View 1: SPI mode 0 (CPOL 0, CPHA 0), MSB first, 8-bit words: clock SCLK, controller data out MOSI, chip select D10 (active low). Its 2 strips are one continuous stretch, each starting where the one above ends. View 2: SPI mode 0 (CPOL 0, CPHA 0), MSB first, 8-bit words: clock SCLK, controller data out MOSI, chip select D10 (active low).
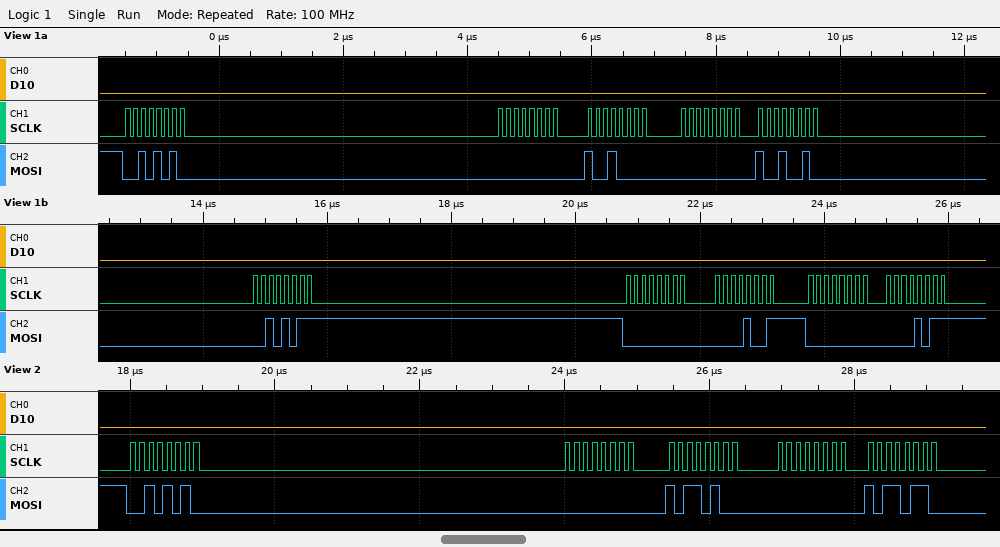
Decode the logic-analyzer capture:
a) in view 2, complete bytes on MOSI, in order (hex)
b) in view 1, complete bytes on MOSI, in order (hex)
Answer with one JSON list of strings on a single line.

["2A 00 B4 00 B6", "0x2A 0x00 0x90 0x00 0x92 0x2B 0x00 0x09 0x00 0x0B"]
